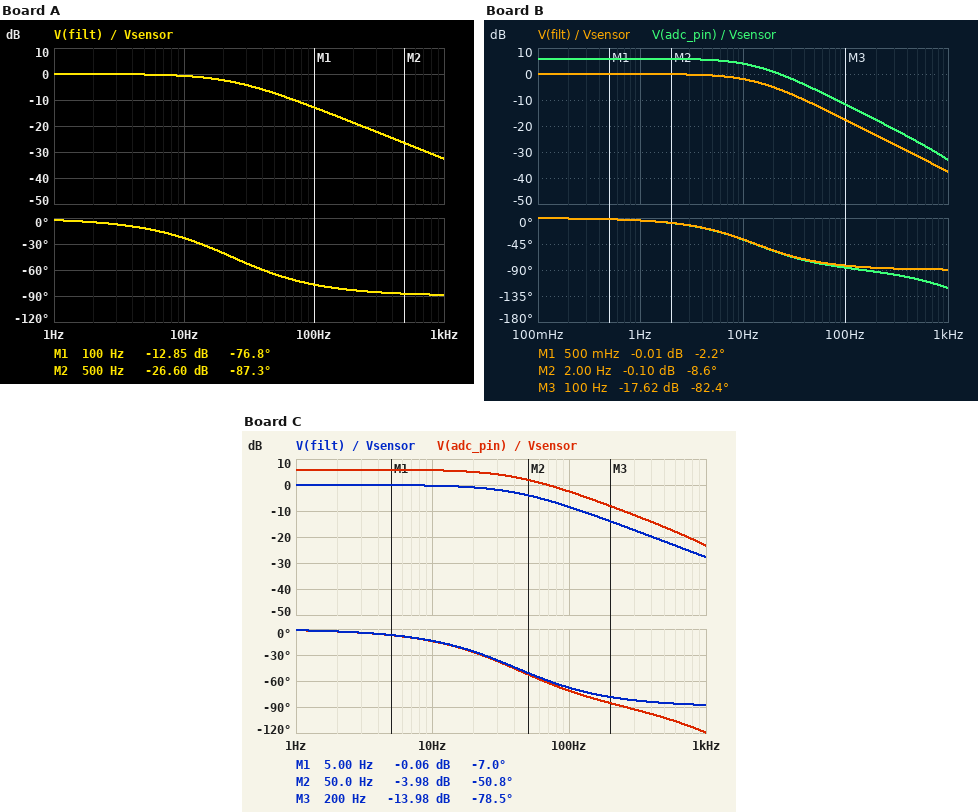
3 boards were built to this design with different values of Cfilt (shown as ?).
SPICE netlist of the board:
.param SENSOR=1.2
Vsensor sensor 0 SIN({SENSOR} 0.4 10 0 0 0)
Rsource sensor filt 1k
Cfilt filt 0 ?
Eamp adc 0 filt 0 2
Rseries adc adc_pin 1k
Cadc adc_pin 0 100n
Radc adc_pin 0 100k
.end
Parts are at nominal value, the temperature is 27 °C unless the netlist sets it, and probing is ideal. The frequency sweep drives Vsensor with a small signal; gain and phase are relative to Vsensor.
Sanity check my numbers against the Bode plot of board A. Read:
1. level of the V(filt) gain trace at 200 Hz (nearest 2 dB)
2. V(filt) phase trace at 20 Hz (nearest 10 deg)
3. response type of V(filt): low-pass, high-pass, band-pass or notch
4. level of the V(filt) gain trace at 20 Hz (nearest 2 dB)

-18 dB
-40 deg
low-pass
-2 dB
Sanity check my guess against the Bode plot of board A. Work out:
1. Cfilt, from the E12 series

6.8 µF
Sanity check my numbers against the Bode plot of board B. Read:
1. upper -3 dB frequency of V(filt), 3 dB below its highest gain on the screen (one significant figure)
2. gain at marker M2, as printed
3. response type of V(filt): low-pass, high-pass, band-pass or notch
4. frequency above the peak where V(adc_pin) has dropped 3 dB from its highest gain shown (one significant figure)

10 Hz
-0.10 dB
low-pass
10 Hz
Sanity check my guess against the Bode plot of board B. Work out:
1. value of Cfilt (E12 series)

12 µF
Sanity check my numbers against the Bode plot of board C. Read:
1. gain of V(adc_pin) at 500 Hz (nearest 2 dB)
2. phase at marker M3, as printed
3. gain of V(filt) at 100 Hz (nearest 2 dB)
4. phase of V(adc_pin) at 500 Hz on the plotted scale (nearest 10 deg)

-16 dB
-78.5 deg
-8 dB
-100 deg
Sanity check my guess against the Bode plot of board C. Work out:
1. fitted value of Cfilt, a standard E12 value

3.9 µF
